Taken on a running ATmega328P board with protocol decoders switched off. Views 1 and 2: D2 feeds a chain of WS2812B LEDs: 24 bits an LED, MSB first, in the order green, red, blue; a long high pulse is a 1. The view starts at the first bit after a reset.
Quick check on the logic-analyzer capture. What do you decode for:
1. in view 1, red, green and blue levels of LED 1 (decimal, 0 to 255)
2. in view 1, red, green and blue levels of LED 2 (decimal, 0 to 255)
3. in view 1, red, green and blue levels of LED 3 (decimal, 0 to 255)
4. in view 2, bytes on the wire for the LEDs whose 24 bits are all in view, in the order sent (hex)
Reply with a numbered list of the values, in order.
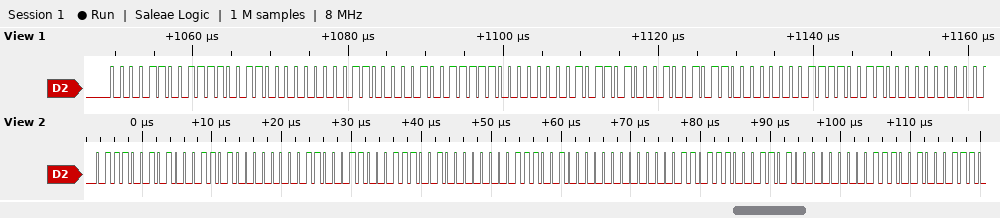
1. 243, 12, 0
2. 159, 96, 0
3. 75, 180, 0
4. 72 8D 00 C6 39 00 E4 00 1B 8D 00 72
